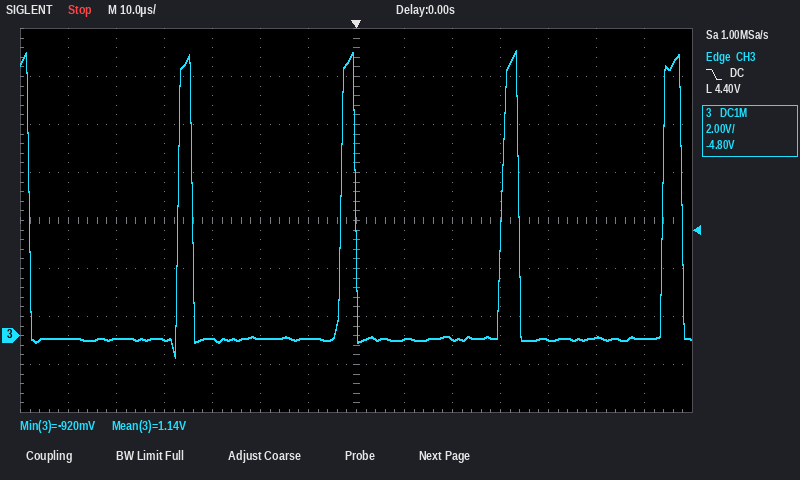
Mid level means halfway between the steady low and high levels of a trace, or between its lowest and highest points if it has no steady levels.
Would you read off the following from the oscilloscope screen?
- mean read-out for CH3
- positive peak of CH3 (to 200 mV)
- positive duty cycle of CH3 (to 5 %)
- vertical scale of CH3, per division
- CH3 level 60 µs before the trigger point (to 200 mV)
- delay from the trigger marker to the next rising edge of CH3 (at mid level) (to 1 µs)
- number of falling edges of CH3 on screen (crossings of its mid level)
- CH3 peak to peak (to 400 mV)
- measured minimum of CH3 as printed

1.14 V
11.8 V
10 %
2 V
-200 mV
30 µs
5
12.8 V
-920 mV
